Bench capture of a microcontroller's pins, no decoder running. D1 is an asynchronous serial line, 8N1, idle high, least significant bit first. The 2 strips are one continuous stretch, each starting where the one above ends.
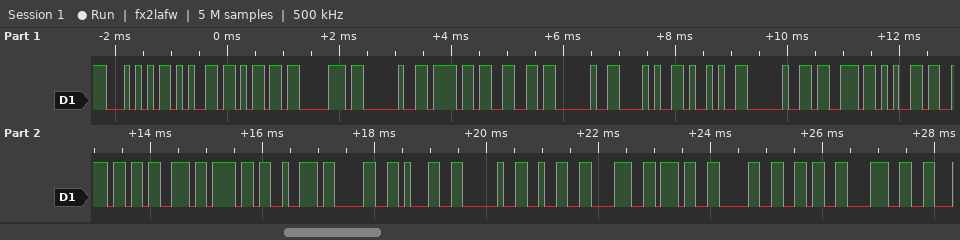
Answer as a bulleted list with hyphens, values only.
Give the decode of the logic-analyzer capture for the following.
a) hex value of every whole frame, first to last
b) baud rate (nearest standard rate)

- 54 65 6D 70 20 6F 66 20 28 29 20 73 65 6E 73 6F 72 30 31 20 32 38 37 30 36 38
- 9600 baud
